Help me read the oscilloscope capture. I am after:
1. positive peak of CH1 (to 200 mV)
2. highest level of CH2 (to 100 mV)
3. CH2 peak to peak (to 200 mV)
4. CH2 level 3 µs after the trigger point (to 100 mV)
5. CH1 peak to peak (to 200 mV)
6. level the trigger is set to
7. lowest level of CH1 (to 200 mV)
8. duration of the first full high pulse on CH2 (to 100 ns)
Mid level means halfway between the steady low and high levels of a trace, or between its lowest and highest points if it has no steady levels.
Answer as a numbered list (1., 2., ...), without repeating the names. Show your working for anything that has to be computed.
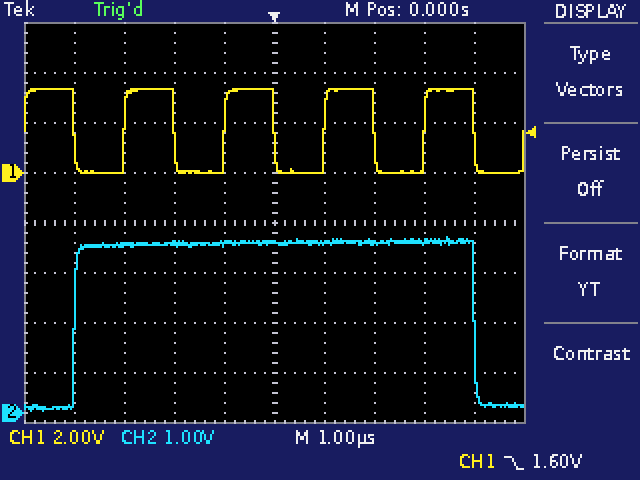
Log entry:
1. 3.4 V
2. 3.5 V
3. 3.4 V
4. 3.4 V
5. 3.4 V − (0.0 V) = 3.4 V
6. 1.60 V
7. 0.0 V
8. 8.0 µs
